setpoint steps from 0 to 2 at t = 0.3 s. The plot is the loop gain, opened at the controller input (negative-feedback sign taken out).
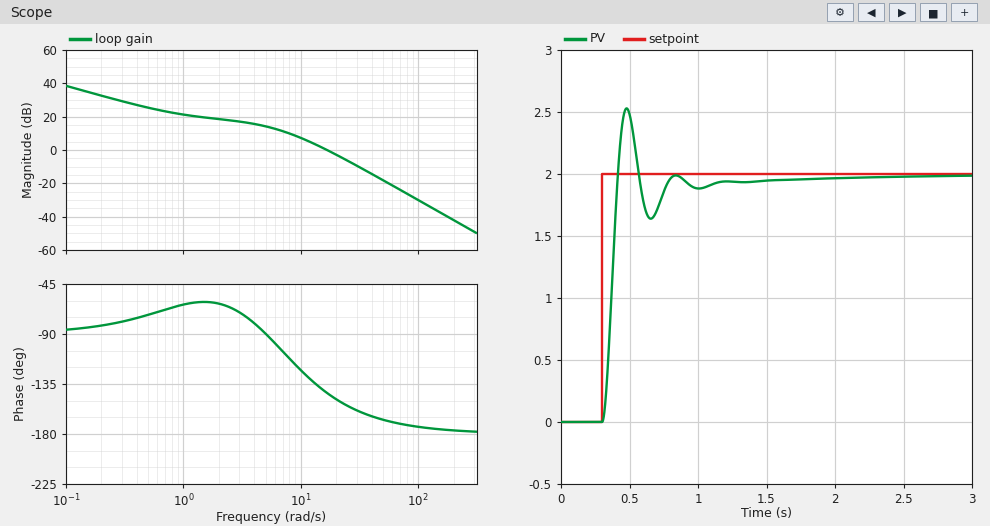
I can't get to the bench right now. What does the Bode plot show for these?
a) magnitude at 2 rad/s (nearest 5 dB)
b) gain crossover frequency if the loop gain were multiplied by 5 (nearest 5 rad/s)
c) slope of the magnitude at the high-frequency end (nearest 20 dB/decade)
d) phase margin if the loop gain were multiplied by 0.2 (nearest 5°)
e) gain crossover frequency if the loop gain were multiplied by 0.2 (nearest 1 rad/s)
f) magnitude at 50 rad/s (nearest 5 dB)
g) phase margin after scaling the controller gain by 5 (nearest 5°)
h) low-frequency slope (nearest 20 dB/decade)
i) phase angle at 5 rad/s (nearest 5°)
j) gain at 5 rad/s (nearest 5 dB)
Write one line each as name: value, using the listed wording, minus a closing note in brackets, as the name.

magnitude at 2 rad/s: 20 dB
gain crossover frequency if the loop gain were multiplied by 5: 40 rad/s
slope of the magnitude at the high-frequency end: -40 dB/decade
phase margin if the loop gain were multiplied by 0.2: 90°
gain crossover frequency if the loop gain were multiplied by 0.2: 5 rad/s
magnitude at 50 rad/s: -20 dB
phase margin after scaling the controller gain by 5: 15°
low-frequency slope: -20 dB/decade
phase angle at 5 rad/s: -90°
gain at 5 rad/s: 15 dB
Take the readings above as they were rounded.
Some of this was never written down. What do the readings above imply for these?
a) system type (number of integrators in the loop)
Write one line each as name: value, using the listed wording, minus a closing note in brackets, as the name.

system type: 1
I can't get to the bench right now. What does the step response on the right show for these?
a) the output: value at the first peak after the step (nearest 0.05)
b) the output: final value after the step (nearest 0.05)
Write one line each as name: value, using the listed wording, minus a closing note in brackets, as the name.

the output: value at the first peak after the step: 2.55
the output: final value after the step: 2.00
